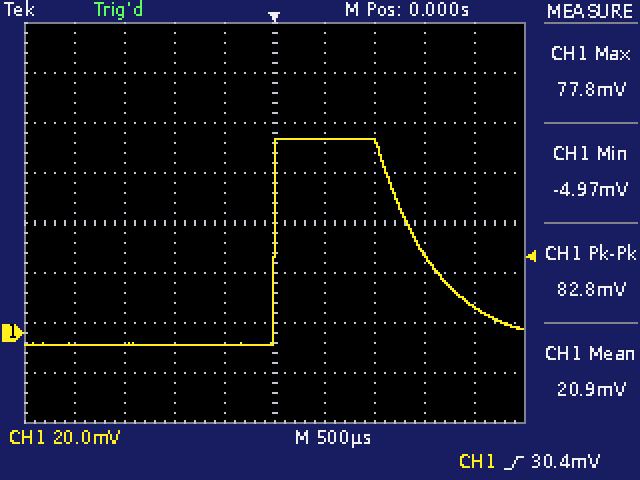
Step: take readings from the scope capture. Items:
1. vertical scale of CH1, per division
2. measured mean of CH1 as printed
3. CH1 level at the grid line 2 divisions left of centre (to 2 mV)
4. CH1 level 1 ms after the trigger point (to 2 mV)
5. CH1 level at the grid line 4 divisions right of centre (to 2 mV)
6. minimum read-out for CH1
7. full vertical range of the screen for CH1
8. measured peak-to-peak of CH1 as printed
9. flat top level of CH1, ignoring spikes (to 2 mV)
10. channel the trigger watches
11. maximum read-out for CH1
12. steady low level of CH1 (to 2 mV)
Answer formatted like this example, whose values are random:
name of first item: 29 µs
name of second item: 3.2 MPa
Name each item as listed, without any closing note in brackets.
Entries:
vertical scale of CH1, per division: 20 mV
measured mean of CH1 as printed: 20.9 mV
CH1 level at the grid line 2 divisions left of centre: -4 mV
CH1 level 1 ms after the trigger point: 76 mV
CH1 level at the grid line 4 divisions right of centre: 10 mV
minimum read-out for CH1: -4.97 mV
full vertical range of the screen for CH1: 160 mV
measured peak-to-peak of CH1 as printed: 82.8 mV
flat top level of CH1, ignoring spikes: 78 mV
channel the trigger watches: CH1
maximum read-out for CH1: 77.8 mV
steady low level of CH1: -4 mV
